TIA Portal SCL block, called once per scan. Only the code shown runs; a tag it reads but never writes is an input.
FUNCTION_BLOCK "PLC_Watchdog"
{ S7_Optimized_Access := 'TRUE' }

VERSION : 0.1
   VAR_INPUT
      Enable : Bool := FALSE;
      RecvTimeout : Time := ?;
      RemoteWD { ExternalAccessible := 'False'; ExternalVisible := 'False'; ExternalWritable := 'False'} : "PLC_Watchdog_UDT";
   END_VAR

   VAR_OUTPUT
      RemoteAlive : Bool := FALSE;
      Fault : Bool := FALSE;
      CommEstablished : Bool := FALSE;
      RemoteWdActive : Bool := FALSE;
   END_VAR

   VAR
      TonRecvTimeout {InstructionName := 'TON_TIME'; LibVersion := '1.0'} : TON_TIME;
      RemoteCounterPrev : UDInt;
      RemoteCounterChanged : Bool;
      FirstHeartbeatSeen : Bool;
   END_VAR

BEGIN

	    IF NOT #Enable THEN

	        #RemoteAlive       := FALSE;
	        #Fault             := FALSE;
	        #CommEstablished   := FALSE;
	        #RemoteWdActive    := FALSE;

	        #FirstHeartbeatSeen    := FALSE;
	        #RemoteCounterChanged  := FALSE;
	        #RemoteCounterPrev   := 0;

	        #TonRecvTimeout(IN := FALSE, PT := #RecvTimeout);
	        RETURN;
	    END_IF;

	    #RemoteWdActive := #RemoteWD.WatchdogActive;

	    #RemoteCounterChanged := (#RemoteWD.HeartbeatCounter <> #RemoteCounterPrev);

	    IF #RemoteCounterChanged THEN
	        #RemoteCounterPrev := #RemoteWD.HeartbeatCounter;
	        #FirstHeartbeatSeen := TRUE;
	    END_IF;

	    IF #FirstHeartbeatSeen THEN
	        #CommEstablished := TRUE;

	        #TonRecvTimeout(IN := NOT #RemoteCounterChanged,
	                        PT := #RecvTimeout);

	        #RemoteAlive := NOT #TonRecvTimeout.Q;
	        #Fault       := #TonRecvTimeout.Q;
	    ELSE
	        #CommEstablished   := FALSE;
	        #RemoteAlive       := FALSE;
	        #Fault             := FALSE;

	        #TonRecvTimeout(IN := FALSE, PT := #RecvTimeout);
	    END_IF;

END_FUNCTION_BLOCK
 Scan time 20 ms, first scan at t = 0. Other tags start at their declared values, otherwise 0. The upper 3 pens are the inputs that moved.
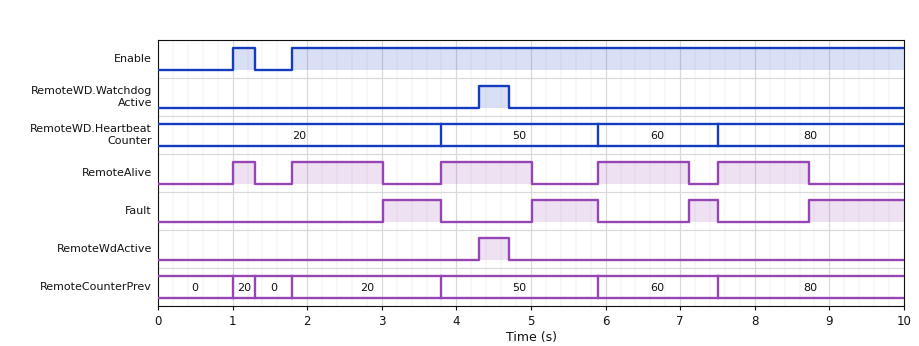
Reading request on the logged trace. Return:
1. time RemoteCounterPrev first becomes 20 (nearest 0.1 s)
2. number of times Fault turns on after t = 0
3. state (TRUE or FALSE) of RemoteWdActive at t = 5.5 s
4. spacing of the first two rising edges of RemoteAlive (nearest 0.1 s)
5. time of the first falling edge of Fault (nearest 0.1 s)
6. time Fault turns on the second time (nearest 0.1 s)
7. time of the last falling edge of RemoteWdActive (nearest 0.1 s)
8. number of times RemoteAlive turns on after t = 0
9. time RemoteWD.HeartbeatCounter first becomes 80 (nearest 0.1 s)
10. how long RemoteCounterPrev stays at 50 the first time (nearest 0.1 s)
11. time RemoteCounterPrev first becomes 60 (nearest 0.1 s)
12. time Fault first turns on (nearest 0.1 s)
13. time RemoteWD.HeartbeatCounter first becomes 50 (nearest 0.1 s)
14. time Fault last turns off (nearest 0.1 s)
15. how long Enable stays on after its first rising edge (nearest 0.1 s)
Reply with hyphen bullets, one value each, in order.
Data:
- 1.0 s
- 4
- FALSE
- 0.8 s
- 3.8 s
- 5.0 s
- 4.7 s
- 5
- 7.5 s
- 2.1 s
- 5.9 s
- 3.0 s
- 3.8 s
- 7.5 s
- 0.3 s
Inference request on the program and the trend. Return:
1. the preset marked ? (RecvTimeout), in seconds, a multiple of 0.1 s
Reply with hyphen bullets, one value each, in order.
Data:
- 1.2 s
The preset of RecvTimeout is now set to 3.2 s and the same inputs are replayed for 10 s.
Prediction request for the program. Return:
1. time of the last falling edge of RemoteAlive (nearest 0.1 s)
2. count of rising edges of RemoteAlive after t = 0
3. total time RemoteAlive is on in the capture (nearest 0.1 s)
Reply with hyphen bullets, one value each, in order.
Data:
- 1.3 s
- 2
- 8.5 s
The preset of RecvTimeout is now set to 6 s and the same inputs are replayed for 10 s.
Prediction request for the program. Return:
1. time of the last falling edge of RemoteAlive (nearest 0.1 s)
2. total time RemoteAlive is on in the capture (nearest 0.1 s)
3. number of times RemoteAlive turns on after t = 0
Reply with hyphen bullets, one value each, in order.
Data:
- 1.3 s
- 8.5 s
- 2
